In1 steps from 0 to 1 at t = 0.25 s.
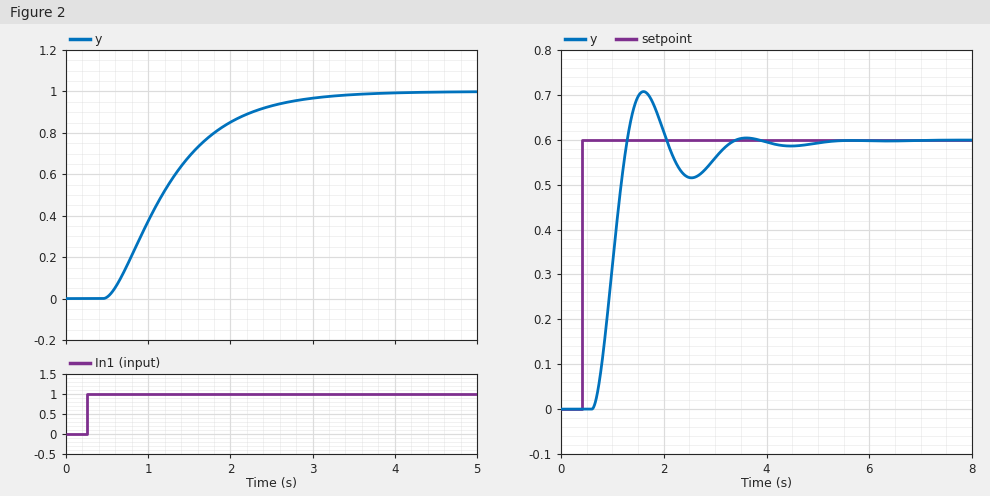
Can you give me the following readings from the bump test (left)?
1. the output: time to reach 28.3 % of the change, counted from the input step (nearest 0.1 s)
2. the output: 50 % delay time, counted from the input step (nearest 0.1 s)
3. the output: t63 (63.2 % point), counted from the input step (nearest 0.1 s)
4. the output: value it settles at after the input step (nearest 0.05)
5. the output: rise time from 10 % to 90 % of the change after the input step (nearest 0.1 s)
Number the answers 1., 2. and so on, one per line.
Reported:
1. 0.6 s
2. 0.9 s
3. 1.1 s
4. 1.00
5. 1.6 s
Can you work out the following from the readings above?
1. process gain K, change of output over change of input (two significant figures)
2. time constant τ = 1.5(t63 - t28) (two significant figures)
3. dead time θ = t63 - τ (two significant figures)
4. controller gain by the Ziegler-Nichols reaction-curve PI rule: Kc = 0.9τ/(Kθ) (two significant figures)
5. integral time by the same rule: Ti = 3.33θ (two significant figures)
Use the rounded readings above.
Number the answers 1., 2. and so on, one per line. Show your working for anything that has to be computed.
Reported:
1. (1 - 0) / 1 = 1.0
2. 1.5 × (1.1 - 0.6) = 0.75 s
3. 1.1 - 0.75 = 0.35 s
4. 0.9 × 0.75 / (1 × 0.35) = 1.9
5. 3.33 × 0.35 = 1.2 s
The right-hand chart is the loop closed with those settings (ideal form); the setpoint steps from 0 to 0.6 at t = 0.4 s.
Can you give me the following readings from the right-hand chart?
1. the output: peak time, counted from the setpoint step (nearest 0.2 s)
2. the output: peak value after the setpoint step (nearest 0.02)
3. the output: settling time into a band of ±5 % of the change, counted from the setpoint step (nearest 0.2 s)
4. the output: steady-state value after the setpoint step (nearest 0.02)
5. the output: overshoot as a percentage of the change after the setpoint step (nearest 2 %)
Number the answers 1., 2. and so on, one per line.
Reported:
1. 1.2 s
2. 0.70
3. 2.6 s
4. 0.60
5. 18 %
